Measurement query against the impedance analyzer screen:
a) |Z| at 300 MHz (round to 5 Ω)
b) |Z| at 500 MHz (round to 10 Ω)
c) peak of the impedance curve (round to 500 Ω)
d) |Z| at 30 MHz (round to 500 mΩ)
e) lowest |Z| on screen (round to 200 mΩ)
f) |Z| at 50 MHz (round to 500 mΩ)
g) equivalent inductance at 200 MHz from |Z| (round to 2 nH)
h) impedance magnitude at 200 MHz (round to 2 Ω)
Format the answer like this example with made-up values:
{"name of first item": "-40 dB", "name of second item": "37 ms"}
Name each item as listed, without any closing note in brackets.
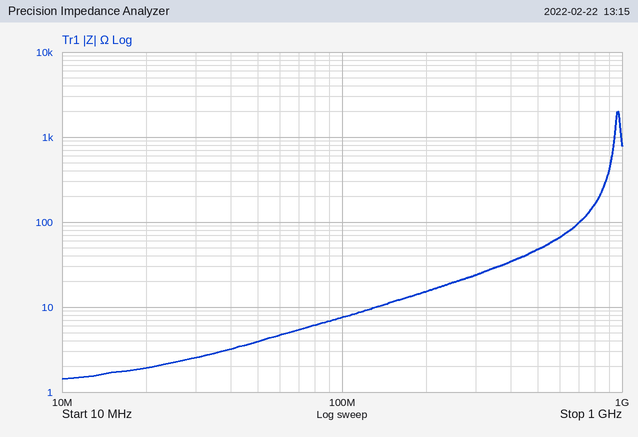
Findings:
{"|Z| at 300 MHz": "25 Ω", "|Z| at 500 MHz": "50 Ω", "peak of the impedance curve": "2.0 kΩ", "|Z| at 30 MHz": "2.5 Ω", "lowest |Z| on screen": "1.4 Ω", "|Z| at 50 MHz": "4.0 Ω", "equivalent inductance at 200 MHz from |Z|": "12 nH", "impedance magnitude at 200 MHz": "16 Ω"}
